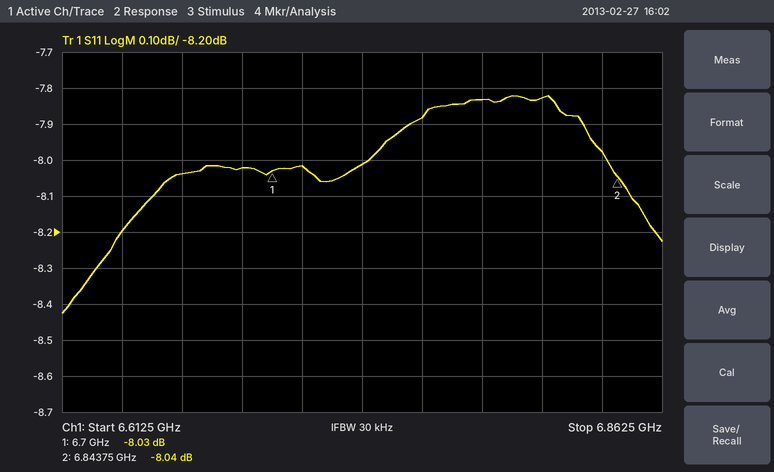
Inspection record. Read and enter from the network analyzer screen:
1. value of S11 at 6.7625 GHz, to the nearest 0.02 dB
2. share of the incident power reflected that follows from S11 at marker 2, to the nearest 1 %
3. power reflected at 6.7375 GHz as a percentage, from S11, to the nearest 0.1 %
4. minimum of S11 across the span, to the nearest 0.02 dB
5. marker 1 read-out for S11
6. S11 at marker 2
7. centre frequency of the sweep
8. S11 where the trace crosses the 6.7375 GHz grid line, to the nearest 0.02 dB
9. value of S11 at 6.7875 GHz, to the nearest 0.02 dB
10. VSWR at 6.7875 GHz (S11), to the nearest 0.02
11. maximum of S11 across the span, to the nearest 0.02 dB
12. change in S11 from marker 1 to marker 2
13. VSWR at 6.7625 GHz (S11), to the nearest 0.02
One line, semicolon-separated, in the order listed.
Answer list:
-7.88 dB; 16 %; 15.8 %; -8.42 dB; -8.03 dB; -8.04 dB; 6.7375 GHz; -8.02 dB; -7.84 dB; 2.36; -7.82 dB; -0.01 dB; 2.36
